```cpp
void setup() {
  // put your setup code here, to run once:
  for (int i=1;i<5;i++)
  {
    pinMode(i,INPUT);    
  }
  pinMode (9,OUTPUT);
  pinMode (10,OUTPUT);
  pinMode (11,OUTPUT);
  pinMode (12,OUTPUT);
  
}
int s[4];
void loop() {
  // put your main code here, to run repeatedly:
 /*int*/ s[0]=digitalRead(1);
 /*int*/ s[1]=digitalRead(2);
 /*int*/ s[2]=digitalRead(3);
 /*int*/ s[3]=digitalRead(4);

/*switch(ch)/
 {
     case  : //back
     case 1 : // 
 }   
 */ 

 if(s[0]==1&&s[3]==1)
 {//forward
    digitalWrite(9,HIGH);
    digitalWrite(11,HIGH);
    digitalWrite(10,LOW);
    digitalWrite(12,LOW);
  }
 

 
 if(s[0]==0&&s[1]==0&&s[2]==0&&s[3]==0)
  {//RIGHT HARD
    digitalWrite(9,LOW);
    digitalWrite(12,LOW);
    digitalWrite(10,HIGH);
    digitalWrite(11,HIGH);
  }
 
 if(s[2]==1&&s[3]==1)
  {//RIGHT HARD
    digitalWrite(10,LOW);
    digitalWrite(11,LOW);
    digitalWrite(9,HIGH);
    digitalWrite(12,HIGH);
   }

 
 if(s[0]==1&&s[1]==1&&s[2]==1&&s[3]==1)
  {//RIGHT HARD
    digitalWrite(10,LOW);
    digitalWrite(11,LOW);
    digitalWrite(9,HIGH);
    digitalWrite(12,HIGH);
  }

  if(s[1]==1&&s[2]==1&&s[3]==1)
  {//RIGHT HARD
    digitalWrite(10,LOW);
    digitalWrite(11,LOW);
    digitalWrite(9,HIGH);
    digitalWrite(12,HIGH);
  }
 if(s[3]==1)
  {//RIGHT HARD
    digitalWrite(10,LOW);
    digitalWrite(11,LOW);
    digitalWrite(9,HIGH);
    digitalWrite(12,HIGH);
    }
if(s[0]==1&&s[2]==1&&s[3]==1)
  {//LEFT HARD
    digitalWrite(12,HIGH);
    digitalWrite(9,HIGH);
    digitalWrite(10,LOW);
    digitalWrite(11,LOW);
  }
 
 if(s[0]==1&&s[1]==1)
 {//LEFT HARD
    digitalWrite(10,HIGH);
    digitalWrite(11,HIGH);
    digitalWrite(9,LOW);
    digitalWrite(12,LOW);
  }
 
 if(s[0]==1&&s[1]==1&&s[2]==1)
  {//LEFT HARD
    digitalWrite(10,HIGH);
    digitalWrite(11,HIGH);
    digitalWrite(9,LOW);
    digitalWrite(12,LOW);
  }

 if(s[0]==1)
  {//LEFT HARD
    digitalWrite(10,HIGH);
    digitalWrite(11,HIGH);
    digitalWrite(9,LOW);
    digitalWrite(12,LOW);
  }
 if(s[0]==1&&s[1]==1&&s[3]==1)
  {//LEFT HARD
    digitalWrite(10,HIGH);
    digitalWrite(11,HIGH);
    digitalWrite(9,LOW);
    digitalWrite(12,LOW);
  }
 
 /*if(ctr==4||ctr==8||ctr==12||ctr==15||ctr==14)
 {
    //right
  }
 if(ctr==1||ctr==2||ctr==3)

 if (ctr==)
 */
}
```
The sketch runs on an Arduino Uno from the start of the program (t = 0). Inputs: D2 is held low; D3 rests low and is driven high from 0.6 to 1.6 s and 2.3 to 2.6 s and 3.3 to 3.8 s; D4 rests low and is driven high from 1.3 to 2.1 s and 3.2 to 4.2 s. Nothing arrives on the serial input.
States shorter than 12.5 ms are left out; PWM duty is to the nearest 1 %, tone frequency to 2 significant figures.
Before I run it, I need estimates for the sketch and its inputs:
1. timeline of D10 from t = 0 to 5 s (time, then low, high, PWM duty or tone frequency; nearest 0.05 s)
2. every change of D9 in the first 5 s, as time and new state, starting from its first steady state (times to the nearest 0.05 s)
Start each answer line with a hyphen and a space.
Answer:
- 0 s high; 1.3 s low; 2.1 s high; 3.2 s low; 4.2 s high
- 0 s low; 1.3 s high; 2.1 s low; 3.2 s high; 4.2 s low
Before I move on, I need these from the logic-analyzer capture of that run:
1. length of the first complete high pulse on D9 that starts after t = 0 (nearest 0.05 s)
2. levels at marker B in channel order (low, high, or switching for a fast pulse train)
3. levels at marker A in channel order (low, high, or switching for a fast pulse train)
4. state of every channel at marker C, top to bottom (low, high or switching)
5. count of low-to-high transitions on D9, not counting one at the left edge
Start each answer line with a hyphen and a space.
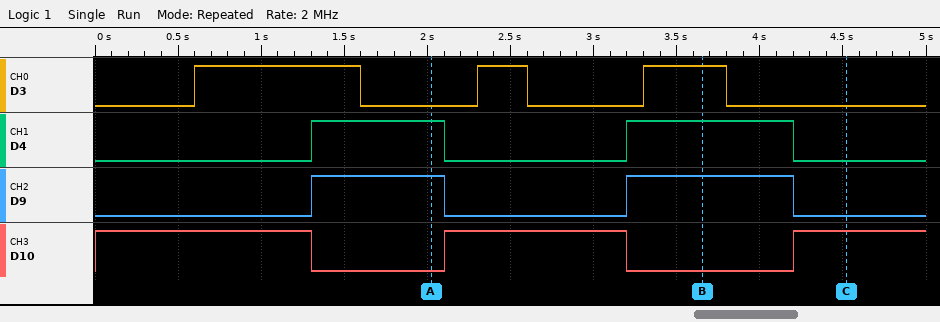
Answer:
- 0.80 s
- D3 high, D4 high, D9 high, D10 low
- D3 low, D4 high, D9 high, D10 low
- D3 low, D4 low, D9 low, D10 high
- 2
